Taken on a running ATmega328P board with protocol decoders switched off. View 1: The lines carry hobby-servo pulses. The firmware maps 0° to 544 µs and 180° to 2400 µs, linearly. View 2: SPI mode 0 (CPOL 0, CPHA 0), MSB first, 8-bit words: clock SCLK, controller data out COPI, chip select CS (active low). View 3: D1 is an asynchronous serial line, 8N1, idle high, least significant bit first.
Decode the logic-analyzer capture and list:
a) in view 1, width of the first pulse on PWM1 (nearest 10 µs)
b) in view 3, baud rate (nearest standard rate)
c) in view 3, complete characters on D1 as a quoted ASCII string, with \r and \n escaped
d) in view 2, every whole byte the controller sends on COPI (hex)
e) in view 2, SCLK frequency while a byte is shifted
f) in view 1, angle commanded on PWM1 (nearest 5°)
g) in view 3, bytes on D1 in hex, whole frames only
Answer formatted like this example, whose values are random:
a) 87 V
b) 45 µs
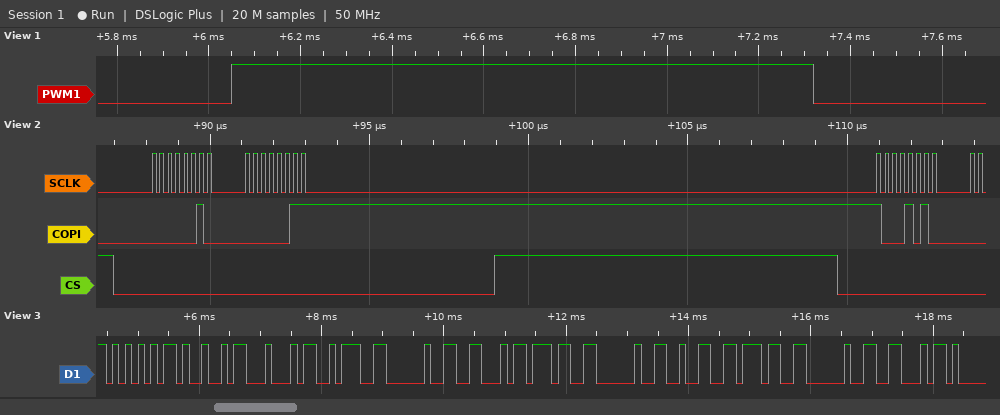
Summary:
a) 1270 µs
b) 9600 baud
c) "UID: F7 27 F"
d) 02 03 8A
e) 4 MHz
f) 70°
g) 55 49 44 3A 20 46 37 20 32 37 20 46
